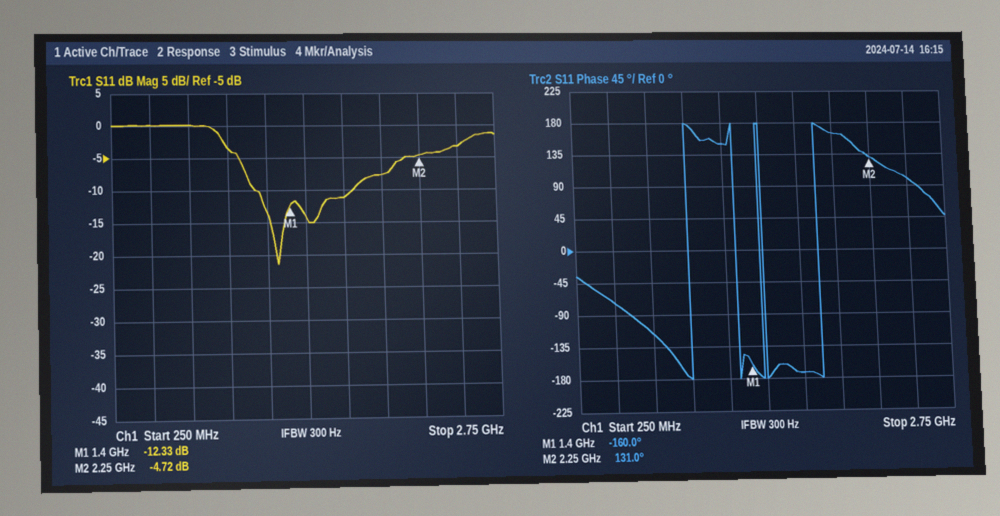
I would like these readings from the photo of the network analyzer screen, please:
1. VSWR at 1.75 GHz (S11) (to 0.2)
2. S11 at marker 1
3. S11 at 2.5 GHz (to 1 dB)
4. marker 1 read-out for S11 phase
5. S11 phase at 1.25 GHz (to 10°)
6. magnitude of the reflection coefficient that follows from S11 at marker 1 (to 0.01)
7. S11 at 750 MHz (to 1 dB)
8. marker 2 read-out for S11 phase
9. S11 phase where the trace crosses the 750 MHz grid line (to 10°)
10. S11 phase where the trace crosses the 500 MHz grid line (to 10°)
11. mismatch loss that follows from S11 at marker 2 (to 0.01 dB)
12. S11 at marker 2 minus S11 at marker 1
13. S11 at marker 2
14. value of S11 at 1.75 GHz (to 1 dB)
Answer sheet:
1.8
-12.33 dB
-3 dB
-160.0°
150°
0.24
0 dB
131.0°
-120°
-70°
1.79 dB
7.61 dB
-4.72 dB
-11 dB
